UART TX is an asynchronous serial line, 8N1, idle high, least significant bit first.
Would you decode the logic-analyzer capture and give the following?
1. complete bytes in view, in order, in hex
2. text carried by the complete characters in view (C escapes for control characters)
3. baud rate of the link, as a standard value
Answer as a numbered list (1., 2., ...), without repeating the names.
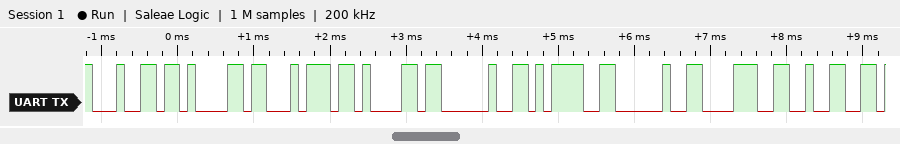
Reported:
1. 0x64 0x61 0x74 0x61 0x20 0x3D 0x20 0x38 0x32
2. "data = 82"
3. 9600 baud
